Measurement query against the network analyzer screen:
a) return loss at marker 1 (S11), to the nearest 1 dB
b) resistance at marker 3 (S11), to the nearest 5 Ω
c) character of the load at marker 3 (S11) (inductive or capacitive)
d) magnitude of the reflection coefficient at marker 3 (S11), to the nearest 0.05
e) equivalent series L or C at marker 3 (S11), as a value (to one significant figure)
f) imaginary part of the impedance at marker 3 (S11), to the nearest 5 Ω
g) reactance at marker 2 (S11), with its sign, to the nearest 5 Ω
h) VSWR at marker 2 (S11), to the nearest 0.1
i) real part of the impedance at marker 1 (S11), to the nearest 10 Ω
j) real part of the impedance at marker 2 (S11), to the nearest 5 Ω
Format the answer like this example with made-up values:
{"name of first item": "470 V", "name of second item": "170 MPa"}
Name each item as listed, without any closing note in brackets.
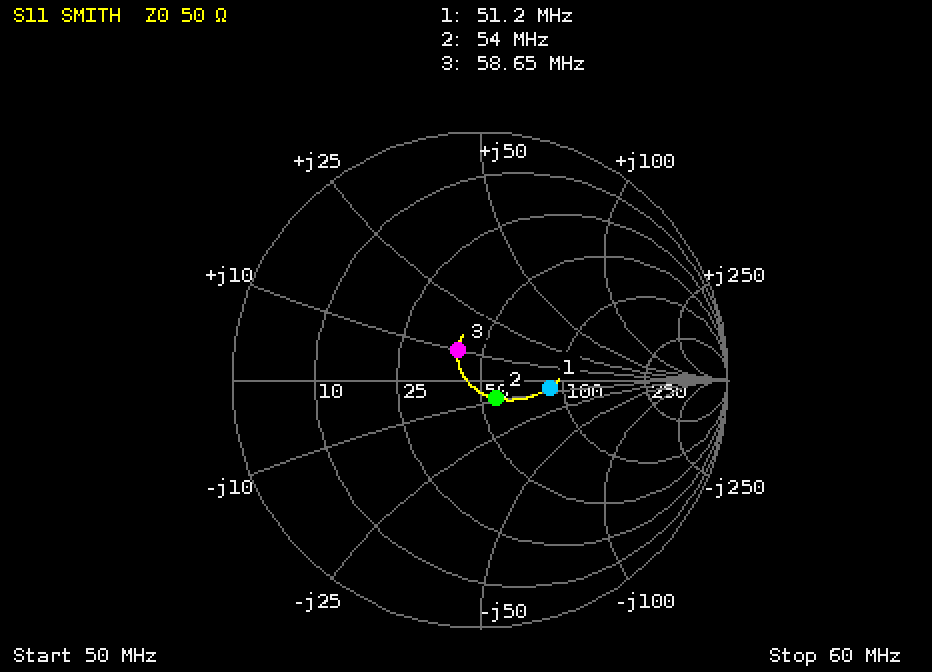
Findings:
{"return loss at marker 1 (S11), to the nearest 1 dB": "11 dB", "resistance at marker 3 (S11), to the nearest 5 Ω": "40 Ω", "character of the load at marker 3 (S11)": "inductive", "magnitude of the reflection coefficient at marker 3 (S11), to the nearest 0.05": "0.15", "equivalent series L or C at marker 3 (S11), as a value": "30 nH", "imaginary part of the impedance at marker 3 (S11), to the nearest 5 Ω": "+10 Ω", "reactance at marker 2 (S11), with its sign, to the nearest 5 Ω": "-10 Ω", "VSWR at marker 2 (S11), to the nearest 0.1": "1.2", "real part of the impedance at marker 1 (S11), to the nearest 10 Ω": "90 Ω", "real part of the impedance at marker 2 (S11), to the nearest 5 Ω": "55 Ω"}
